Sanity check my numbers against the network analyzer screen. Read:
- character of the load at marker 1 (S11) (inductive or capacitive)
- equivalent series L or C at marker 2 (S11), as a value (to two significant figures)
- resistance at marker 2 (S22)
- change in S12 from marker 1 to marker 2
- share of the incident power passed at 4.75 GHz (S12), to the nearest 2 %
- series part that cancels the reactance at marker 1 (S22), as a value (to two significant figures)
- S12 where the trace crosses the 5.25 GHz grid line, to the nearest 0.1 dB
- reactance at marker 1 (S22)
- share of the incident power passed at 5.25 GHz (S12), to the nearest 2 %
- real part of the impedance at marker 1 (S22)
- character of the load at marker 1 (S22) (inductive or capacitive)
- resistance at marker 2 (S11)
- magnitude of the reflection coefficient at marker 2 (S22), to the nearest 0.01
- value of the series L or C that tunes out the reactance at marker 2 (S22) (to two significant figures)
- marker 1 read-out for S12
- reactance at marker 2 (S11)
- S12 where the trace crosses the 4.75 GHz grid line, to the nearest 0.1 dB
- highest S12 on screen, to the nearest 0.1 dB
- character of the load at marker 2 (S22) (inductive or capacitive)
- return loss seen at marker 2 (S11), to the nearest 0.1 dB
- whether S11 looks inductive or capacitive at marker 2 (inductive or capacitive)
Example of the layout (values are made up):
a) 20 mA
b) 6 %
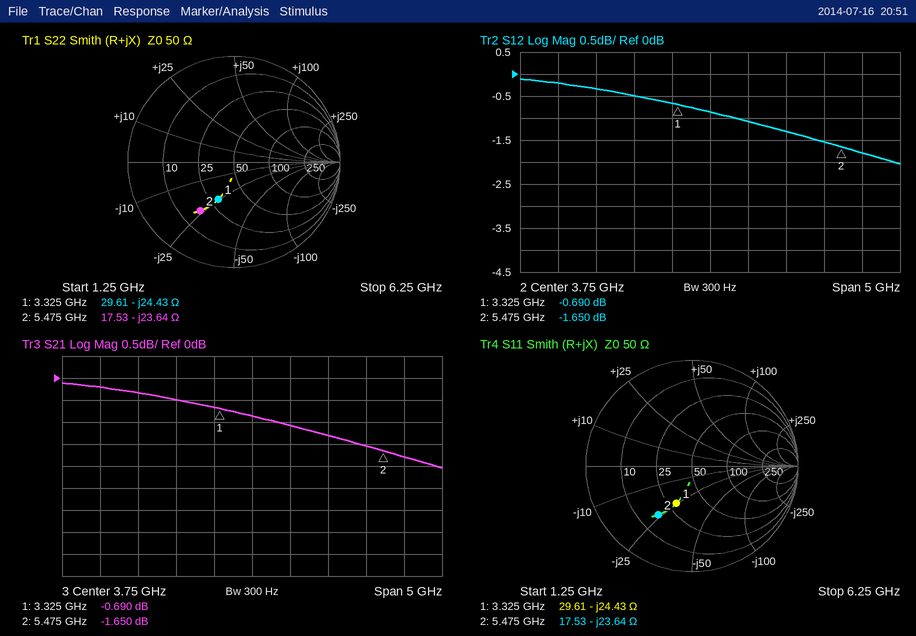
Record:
a) capacitive
b) 1.2 pF
c) 17.53 Ω
d) -0.960 dB
e) 74 %
f) 1.2 nH
g) -1.5 dB
h) -24.43 Ω
i) 70 %
j) 29.61 Ω
k) capacitive
l) 17.53 Ω
m) 0.56
n) 690 pH
o) -0.690 dB
p) -23.64 Ω
q) -1.3 dB
r) -0.1 dB
s) capacitive
t) 5.0 dB
u) capacitive
